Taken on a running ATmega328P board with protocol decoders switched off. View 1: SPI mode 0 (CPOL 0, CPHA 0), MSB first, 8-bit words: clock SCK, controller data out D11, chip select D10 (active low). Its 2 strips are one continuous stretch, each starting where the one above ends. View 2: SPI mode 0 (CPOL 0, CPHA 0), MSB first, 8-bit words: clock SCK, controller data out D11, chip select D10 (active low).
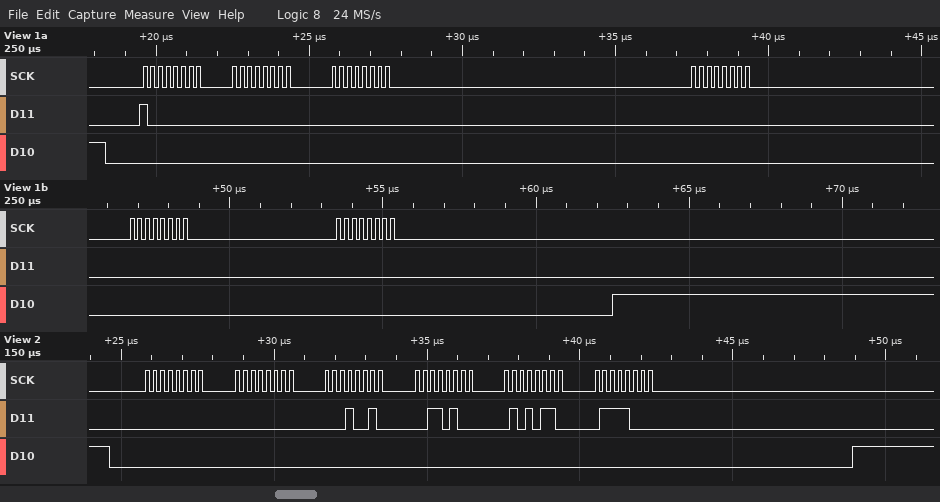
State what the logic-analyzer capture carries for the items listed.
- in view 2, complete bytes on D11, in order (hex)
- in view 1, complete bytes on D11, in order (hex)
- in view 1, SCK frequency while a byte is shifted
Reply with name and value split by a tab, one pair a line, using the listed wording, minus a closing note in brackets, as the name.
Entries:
in view 2, complete bytes on D11, in order	0x00 0x00 0x12 0x34 0x56 0x78
in view 1, complete bytes on D11, in order	80 00 00 00 00 00
in view 1, SCK frequency while a byte is shifted	4 MHz
